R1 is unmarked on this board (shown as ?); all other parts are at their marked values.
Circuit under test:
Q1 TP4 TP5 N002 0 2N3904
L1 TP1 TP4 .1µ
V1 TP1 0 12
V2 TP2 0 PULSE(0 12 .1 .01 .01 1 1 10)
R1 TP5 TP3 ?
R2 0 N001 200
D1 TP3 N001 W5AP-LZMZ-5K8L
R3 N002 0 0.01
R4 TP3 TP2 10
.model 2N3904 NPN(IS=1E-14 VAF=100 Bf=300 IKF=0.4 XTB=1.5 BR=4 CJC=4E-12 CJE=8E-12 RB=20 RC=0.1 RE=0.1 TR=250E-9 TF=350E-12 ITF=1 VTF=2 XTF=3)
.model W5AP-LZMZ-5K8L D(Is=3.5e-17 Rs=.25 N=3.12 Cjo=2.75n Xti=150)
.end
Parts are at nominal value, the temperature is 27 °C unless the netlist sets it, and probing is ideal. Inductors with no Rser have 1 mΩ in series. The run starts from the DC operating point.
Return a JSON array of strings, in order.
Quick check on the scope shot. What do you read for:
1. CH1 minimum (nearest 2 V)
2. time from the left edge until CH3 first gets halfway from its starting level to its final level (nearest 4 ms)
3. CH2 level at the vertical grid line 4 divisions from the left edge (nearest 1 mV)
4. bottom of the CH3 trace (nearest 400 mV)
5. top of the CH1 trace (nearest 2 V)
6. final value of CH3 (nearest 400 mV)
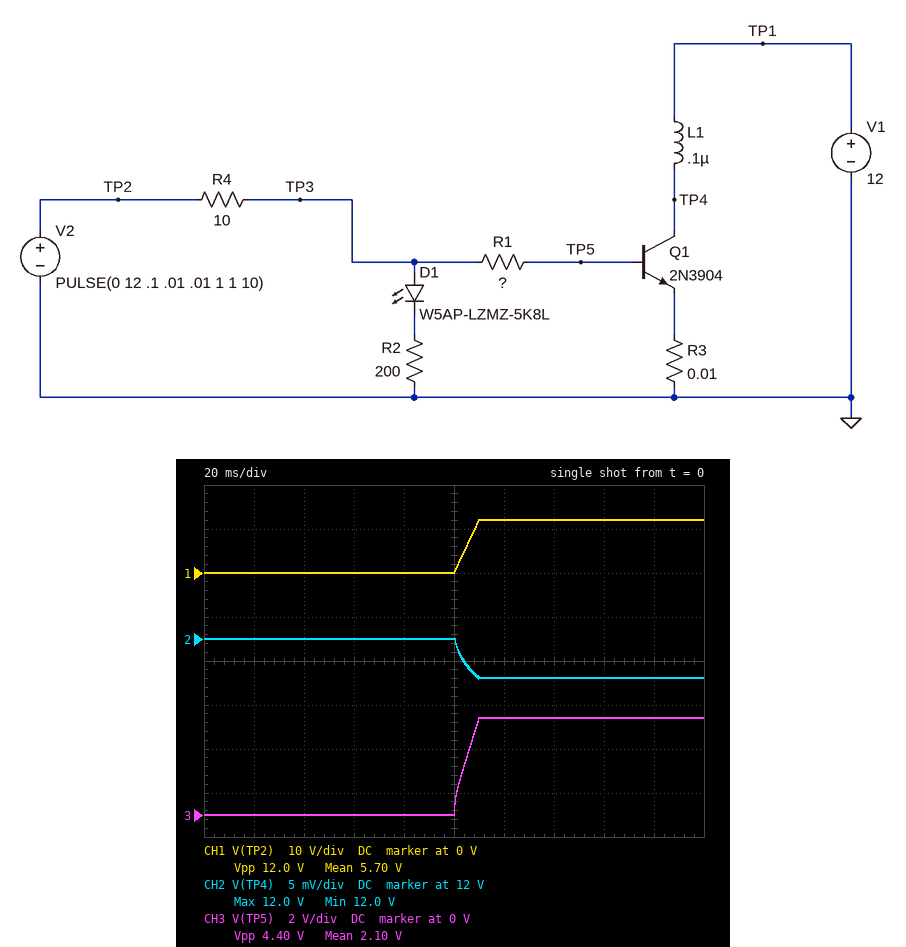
["0 V", "104 ms", "12.000 V", "0 V", "12 V", "4.4 V"]
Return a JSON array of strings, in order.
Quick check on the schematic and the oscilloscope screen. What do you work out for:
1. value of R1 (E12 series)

["39 Ω"]
